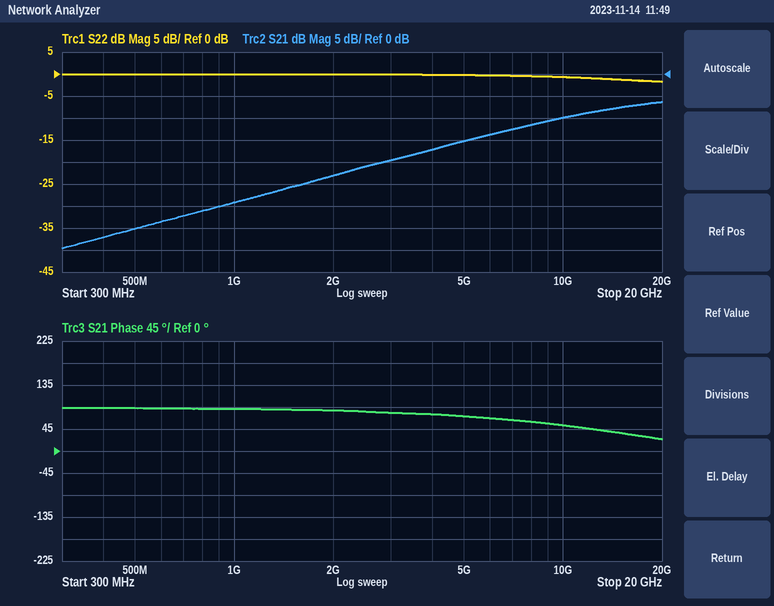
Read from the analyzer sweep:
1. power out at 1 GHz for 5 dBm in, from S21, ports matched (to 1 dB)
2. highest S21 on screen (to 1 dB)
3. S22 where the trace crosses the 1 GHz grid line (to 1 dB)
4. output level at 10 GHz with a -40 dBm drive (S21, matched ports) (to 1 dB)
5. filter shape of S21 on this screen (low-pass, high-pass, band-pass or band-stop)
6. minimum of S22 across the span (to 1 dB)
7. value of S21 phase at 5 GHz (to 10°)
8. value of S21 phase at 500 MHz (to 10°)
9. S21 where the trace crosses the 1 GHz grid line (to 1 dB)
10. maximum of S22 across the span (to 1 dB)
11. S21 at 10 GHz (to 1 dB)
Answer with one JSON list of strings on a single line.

["-24 dBm", "-6 dB", "0 dB", "-50 dBm", "high-pass", "-2 dB", "70°", "90°", "-29 dB", "0 dB", "-10 dB"]
